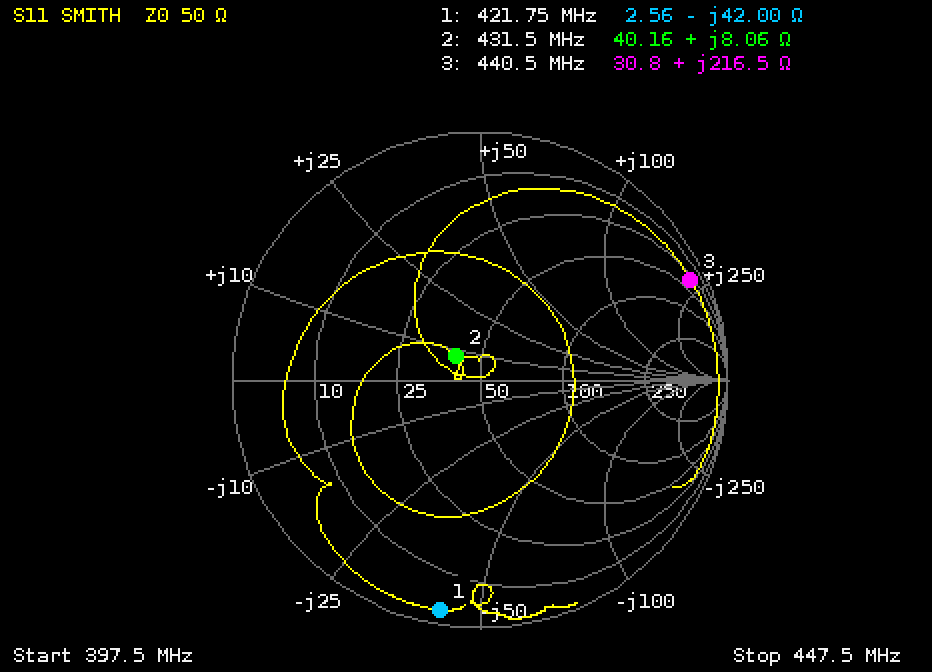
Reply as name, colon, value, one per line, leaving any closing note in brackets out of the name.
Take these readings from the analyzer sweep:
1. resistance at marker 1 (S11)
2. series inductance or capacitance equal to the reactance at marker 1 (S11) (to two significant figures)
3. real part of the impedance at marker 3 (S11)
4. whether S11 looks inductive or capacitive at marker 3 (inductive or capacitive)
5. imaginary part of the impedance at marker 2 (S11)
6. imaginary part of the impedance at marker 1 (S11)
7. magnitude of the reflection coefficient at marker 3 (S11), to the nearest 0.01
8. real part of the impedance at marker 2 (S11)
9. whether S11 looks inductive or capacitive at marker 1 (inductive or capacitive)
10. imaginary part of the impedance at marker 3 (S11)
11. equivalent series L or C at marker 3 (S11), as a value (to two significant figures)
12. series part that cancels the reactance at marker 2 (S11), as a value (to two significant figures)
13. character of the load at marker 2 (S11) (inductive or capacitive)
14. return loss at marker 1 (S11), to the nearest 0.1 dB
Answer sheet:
resistance at marker 1: 2.56 Ω
series inductance or capacitance equal to the reactance at marker 1 (S11): 9.0 pF
real part of the impedance at marker 3: 30.8 Ω
whether S11 looks inductive or capacitive at marker 3: inductive
imaginary part of the impedance at marker 2: +8.06 Ω
imaginary part of the impedance at marker 1: -42.00 Ω
magnitude of the reflection coefficient at marker 3 (S11), to the nearest 0.01: 0.94
real part of the impedance at marker 2: 40.16 Ω
whether S11 looks inductive or capacitive at marker 1: capacitive
imaginary part of the impedance at marker 3: +216.5 Ω
equivalent series L or C at marker 3 (S11), as a value: 78 nH
series part that cancels the reactance at marker 2 (S11), as a value: 46 pF
character of the load at marker 2 (S11): inductive
return loss at marker 1 (S11), to the nearest 0.1 dB: 0.5 dB
